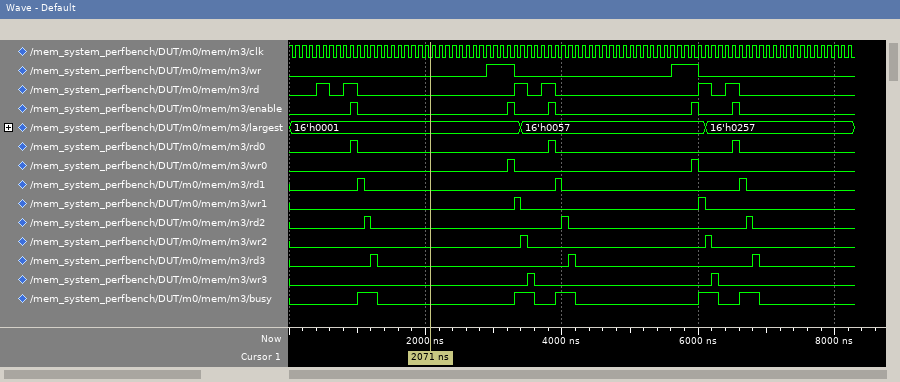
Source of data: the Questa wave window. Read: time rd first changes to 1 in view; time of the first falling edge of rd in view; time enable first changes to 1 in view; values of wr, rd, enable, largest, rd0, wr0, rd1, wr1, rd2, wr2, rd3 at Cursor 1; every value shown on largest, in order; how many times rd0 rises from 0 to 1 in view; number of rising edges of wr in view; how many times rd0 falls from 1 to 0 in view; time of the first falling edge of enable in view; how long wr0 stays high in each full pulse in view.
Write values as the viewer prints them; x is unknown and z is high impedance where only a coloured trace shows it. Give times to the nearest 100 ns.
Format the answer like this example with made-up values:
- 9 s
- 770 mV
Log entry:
- 400 ns
- 600 ns
- 900 ns
- wr=0, rd=0, enable=0, largest=16'h0001, rd0=0, wr0=0, rd1=0, wr1=0, rd2=0, wr2=0, rd3=0
- 16'h0001, 16'h0057, 16'h0257
- 3
- 2
- 3
- 1000 ns
- 100 ns, 100 ns
